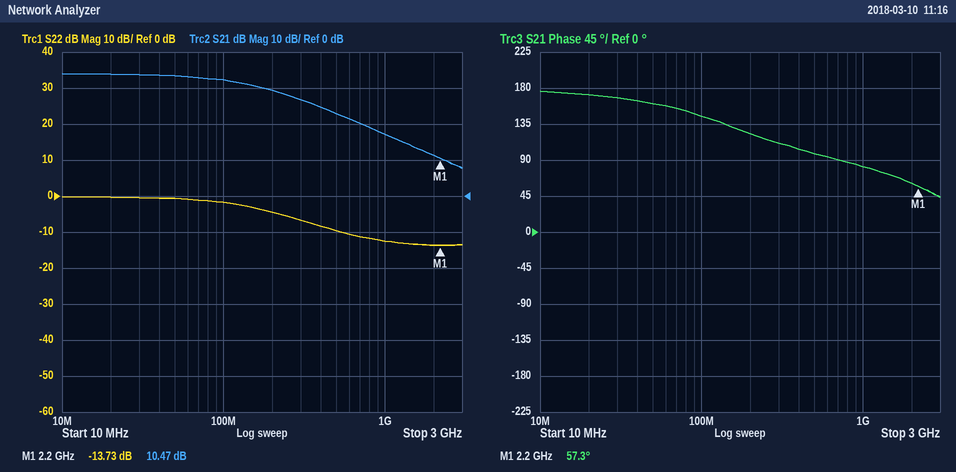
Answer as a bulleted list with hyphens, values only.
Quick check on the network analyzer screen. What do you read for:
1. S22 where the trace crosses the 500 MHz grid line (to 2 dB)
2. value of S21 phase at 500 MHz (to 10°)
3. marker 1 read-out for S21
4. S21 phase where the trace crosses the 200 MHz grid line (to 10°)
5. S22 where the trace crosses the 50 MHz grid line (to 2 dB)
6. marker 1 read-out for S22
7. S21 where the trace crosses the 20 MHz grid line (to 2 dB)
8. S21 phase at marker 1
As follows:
- -10 dB
- 100°
- 10.47 dB
- 120°
- 0 dB
- -13.73 dB
- 34 dB
- 57.3°
